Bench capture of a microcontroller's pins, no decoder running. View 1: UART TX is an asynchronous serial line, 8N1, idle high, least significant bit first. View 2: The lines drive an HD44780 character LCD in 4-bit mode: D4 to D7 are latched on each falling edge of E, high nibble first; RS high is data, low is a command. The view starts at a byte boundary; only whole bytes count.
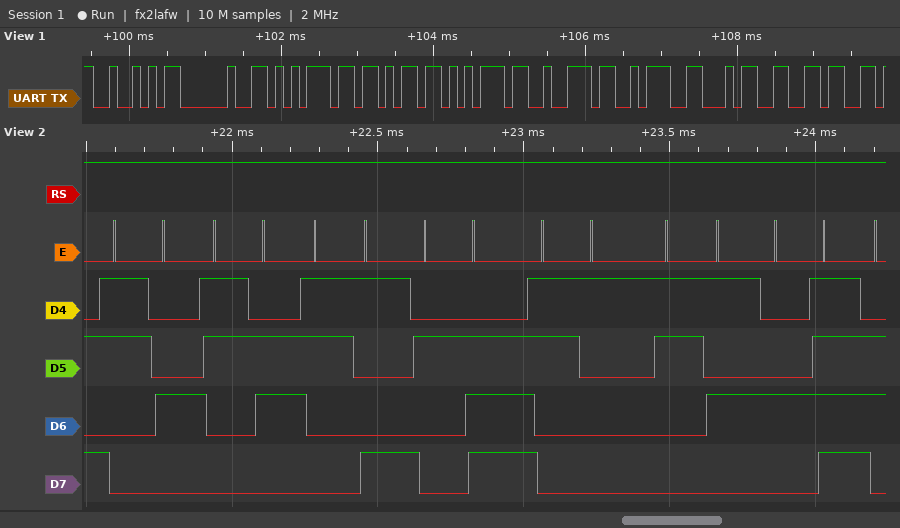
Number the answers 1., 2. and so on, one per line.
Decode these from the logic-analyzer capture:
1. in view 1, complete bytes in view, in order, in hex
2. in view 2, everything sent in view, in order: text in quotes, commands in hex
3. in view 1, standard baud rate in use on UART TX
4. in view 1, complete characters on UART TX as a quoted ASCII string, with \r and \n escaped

1. 52 20 75 6B 75 72 3A 34 36
2. "469.15O"
3. 9600 baud
4. "R ukur:46"
